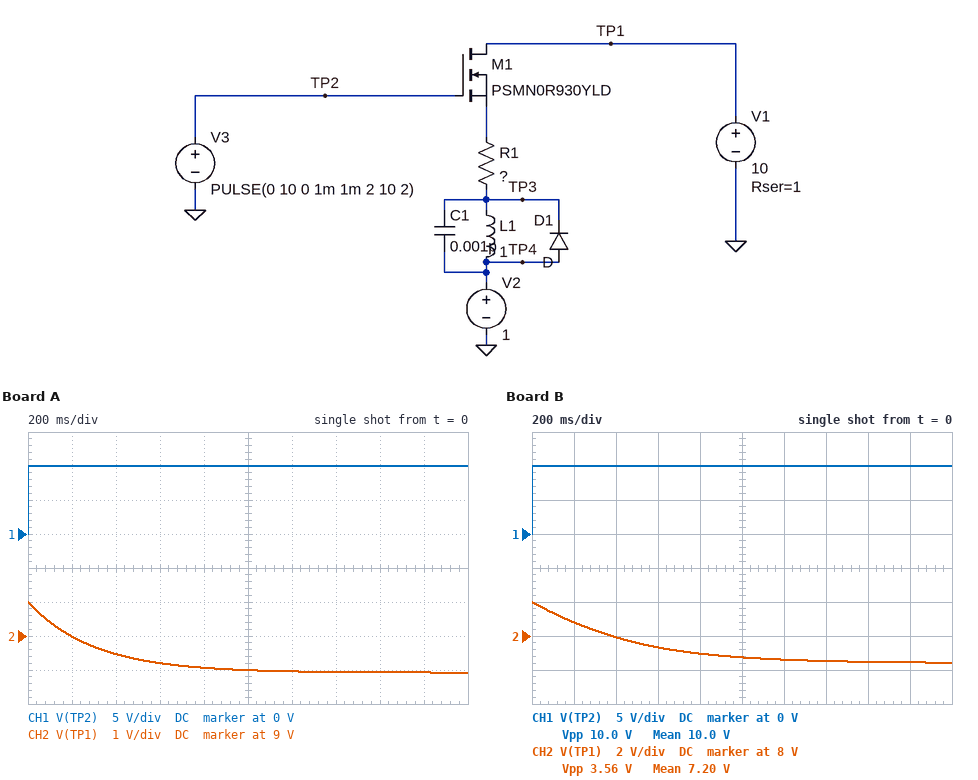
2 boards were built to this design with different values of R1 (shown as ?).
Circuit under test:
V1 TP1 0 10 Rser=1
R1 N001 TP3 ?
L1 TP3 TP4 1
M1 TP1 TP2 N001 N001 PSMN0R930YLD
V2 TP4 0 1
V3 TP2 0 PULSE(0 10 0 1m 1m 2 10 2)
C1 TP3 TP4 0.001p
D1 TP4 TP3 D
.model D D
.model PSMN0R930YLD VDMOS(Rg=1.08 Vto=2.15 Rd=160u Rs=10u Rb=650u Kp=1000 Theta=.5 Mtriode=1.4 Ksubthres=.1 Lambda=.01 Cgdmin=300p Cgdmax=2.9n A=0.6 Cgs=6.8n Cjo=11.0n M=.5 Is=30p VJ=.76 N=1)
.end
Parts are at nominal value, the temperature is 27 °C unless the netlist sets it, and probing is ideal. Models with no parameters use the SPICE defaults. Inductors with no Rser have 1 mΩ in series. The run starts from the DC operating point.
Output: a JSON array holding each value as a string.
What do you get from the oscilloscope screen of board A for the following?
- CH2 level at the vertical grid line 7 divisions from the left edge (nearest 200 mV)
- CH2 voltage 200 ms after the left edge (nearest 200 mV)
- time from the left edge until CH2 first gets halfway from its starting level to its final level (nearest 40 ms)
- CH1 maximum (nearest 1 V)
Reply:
["8.0 V", "9.0 V", "200 ms", "10 V"]
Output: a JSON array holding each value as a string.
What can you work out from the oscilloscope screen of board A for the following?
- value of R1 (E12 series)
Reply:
["3.3 Ω"]
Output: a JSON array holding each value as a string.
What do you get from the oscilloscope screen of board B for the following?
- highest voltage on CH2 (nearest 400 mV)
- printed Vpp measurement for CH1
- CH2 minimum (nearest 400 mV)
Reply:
["10.0 V", "10.0 V", "6.4 V"]
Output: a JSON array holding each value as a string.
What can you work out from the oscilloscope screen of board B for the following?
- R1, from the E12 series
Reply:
["1.5 Ω"]
